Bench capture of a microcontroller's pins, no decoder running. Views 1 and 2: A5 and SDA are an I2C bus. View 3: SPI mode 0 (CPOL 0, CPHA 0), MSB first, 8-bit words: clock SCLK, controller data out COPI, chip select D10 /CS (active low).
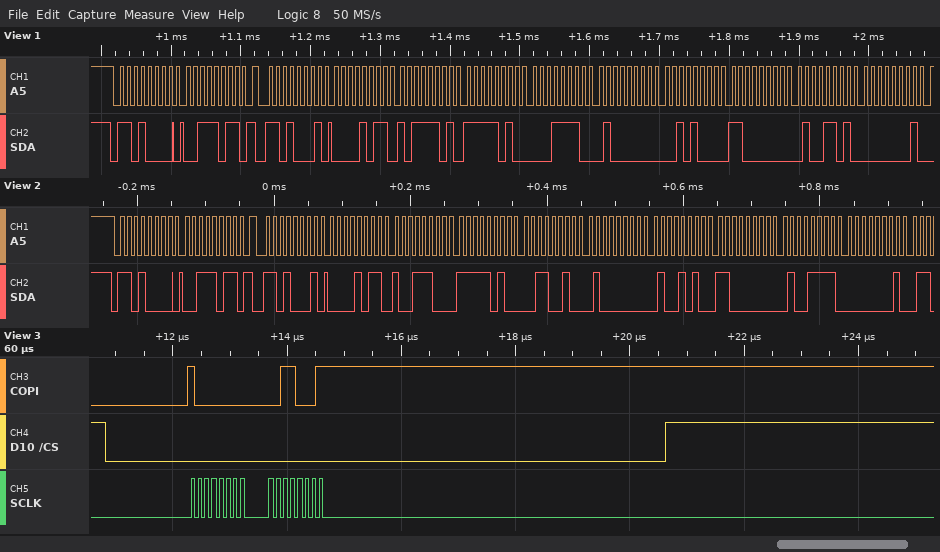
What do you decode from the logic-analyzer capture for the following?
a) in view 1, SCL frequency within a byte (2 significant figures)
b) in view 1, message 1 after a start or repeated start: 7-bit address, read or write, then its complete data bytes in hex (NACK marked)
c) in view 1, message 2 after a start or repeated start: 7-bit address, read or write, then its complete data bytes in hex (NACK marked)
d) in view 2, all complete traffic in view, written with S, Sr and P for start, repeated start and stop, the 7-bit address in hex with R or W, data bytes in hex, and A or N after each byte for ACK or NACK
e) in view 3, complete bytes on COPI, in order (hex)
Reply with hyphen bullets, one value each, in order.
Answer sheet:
- 100 kHz
- 0x68 write: 3B
- 0x68 read: 0B BD FA 1E 40 28 C0 4D 01
- S 68W A 3B A Sr 68R A 0B A 9C A FA A 32 A 40 A 4A A C0 A 4F A 01 A
- 80 31
